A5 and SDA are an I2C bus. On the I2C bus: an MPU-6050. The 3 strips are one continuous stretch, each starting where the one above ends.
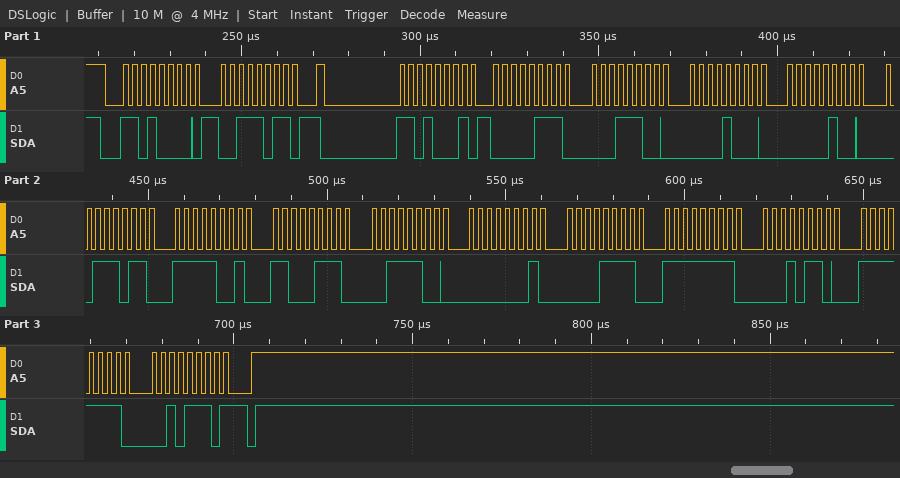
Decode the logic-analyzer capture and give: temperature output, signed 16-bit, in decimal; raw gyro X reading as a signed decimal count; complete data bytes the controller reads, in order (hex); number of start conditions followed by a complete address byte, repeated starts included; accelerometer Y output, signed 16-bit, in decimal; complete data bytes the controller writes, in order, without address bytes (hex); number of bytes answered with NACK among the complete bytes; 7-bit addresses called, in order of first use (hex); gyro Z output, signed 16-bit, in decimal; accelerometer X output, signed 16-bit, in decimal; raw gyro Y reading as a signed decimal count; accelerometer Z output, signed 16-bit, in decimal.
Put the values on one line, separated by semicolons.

-14532; 271; 07 1C 08 04 3B F9 C7 3C 01 0F FF 16 FF 2E; 2; 2052; 3B; 1; 0x68; -210; 1820; -234; 15353
